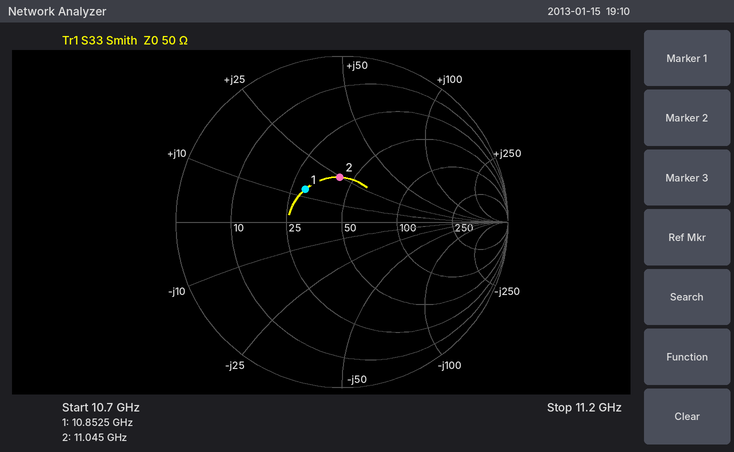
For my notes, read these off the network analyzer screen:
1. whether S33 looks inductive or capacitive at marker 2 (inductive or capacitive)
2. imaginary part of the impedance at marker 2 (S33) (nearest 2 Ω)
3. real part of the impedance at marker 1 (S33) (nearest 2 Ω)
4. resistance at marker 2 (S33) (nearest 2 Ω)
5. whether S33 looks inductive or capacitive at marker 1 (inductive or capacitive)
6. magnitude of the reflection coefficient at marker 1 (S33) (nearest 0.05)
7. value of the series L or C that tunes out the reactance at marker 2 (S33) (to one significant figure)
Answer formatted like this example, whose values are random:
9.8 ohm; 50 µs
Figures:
inductive; +24 Ω; 30 Ω; 42 Ω; inductive; 0.30; 600 fF
